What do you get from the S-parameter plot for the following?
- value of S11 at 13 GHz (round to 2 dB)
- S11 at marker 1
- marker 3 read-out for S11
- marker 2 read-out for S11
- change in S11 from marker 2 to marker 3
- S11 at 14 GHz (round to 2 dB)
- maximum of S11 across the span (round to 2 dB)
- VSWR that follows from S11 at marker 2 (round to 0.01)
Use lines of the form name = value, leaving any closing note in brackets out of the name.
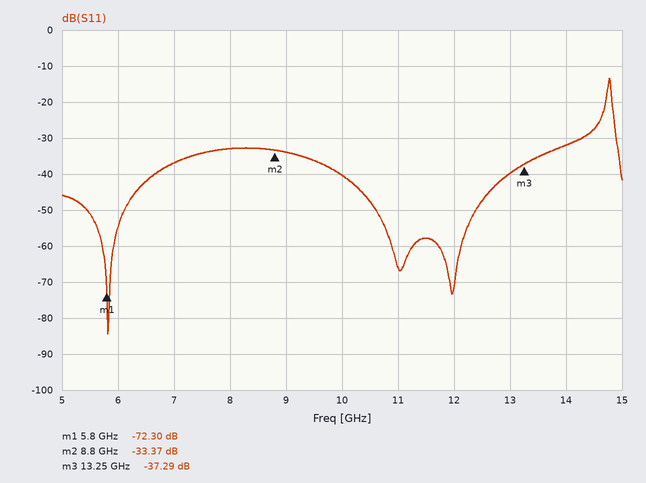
value of S11 at 13 GHz = -40 dB
S11 at marker 1 = -72.30 dB
marker 3 read-out for S11 = -37.29 dB
marker 2 read-out for S11 = -33.37 dB
change in S11 from marker 2 to marker 3 = -3.92 dB
S11 at 14 GHz = -32 dB
maximum of S11 across the span = -14 dB
VSWR that follows from S11 at marker 2 = 1.04
